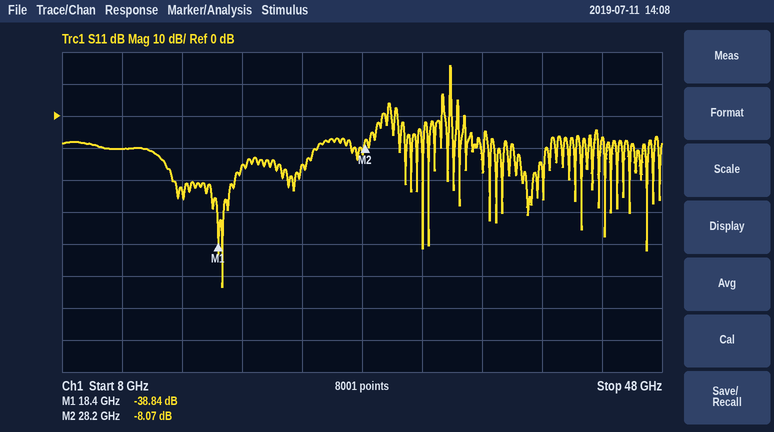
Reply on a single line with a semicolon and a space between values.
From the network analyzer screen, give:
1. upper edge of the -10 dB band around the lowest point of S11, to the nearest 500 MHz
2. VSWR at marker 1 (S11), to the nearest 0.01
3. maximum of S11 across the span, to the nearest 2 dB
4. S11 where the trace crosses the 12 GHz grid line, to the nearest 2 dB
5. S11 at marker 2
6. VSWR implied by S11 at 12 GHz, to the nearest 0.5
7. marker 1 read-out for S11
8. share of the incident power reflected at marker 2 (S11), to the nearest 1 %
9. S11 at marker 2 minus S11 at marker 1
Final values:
25.0 GHz; 1.02; 16 dB; -10 dB; -8.07 dB; 2.0; -38.84 dB; 16 %; 30.77 dB
